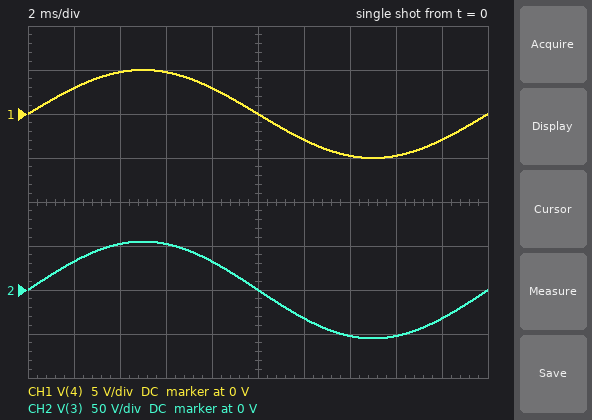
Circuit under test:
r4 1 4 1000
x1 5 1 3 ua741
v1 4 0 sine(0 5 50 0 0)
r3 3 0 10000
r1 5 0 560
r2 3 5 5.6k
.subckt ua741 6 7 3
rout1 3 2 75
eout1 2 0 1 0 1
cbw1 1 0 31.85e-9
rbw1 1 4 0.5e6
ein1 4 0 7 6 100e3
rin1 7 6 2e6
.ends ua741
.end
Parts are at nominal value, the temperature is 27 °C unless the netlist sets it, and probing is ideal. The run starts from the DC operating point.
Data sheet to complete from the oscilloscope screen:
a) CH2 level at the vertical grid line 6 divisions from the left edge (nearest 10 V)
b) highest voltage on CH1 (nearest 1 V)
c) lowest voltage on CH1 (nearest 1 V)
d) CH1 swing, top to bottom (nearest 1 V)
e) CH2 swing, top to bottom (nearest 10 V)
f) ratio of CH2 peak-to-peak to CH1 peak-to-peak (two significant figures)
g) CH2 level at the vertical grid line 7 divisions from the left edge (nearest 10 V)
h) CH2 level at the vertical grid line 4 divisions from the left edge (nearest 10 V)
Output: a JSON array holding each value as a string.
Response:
["-30 V", "5 V", "-5 V", "10 V", "110 V", "11", "-50 V", "30 V"]
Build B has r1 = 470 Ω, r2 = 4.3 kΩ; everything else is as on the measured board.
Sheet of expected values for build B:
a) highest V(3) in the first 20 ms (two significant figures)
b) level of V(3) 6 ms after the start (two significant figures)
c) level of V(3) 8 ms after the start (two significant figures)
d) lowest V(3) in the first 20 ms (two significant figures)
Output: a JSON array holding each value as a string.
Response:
["51 V", "48 V", "30 V", "-51 V"]
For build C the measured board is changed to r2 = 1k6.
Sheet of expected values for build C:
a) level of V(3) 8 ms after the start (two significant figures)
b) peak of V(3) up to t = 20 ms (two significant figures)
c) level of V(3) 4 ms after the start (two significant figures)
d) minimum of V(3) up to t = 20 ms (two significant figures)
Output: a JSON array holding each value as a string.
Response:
["11 V", "19 V", "18 V", "-19 V"]
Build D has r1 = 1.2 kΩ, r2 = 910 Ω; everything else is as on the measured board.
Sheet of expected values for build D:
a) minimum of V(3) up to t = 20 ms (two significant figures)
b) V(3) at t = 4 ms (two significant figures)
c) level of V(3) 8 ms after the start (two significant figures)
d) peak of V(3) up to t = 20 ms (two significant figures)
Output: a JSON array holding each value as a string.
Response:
["-8.8 V", "8.4 V", "5.2 V", "8.8 V"]
